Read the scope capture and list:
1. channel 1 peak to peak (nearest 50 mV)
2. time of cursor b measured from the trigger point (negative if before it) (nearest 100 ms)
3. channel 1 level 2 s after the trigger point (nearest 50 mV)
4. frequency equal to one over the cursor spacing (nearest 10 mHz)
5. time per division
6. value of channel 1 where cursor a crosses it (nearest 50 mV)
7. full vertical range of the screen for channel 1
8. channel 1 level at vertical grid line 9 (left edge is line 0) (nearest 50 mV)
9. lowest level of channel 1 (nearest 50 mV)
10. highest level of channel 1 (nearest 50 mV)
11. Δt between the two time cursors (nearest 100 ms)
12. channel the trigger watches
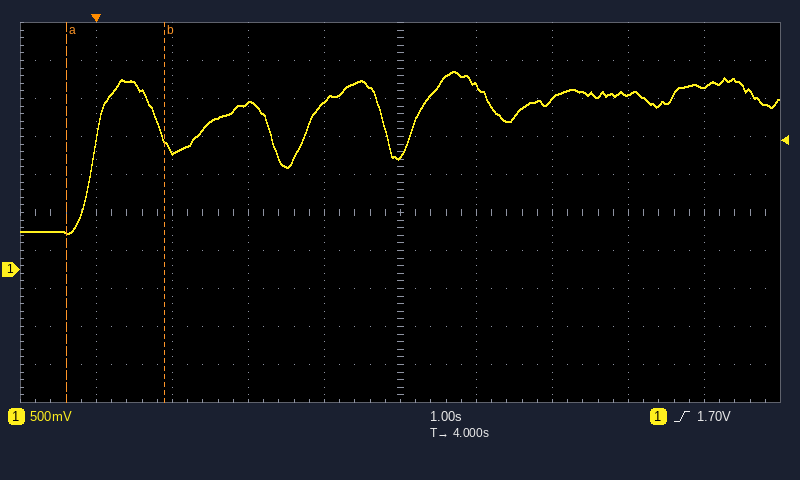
2.15 V
+900 ms
2.20 V
770 mHz
1 s
500 mV
5 V
2.40 V
450 mV
2.60 V
1.3 s
channel 1
